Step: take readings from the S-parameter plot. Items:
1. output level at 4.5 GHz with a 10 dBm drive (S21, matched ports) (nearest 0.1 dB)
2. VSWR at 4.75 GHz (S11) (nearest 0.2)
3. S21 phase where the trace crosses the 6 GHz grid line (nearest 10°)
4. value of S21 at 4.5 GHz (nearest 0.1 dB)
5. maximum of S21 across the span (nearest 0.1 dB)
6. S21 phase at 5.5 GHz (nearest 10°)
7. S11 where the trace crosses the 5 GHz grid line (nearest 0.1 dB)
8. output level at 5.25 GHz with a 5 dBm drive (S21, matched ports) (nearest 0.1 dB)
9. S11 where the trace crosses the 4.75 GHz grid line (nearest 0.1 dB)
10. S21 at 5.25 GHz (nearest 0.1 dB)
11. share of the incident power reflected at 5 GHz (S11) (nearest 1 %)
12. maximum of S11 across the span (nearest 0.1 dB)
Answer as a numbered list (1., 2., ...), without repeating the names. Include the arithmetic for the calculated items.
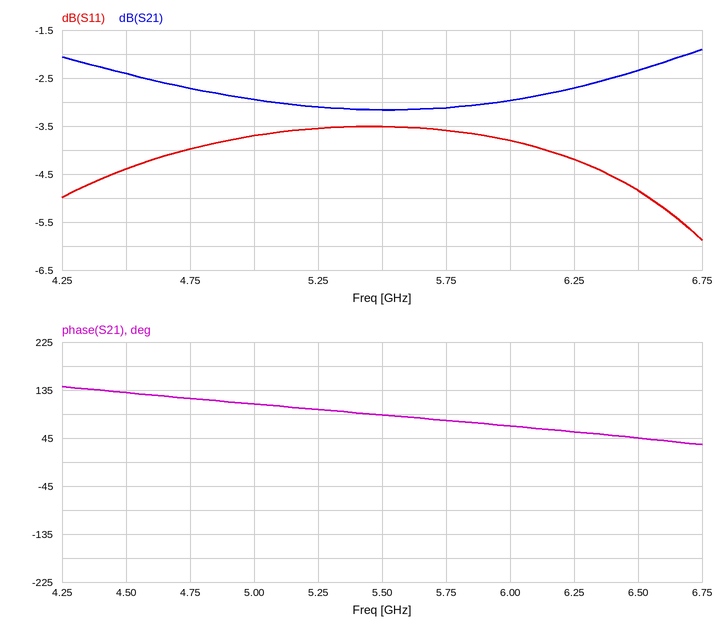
1. 10 dBm + (-2.4 dB) = 7.6 dBm
2. |Γ| = 10^(-4/20) = 0.6310; VSWR = (1 + 0.6310)/(1 − 0.6310) ≈ 4.4
3. 70°
4. -2.4 dB
5. -1.9 dB
6. 90°
7. -3.7 dB
8. 5 dBm + (-3.1 dB) = 1.9 dBm
9. -4.0 dB
10. -3.1 dB
11. 10^(-3.7/10) ≈ 43 %
12. -3.5 dB
